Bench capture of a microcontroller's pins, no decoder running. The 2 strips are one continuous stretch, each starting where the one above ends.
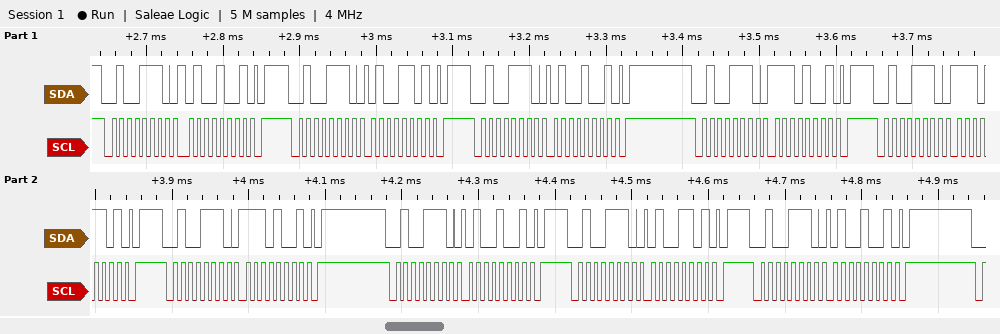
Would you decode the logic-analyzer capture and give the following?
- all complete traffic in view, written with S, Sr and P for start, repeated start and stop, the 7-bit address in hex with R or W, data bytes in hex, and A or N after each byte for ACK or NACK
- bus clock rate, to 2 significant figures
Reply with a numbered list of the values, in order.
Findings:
1. S 27W A 49 A P S 27W A 4D A P S 27W A 49 A P S 27W A E9 A P S 27W A ED A P S 27W A E9 A P S 27W A 49 A P S 27W A 4D A P S 27W A 49 A P
2. 100 kHz
